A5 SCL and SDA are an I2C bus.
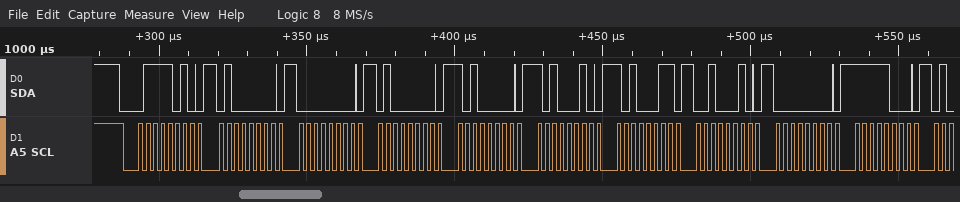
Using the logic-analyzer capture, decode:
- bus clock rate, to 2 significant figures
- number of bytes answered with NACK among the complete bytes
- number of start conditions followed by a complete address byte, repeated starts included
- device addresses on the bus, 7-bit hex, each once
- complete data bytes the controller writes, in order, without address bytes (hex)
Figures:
400 kHz
0
1
0x3D
40 00 40 A0 A2 A3 22 00 F8
